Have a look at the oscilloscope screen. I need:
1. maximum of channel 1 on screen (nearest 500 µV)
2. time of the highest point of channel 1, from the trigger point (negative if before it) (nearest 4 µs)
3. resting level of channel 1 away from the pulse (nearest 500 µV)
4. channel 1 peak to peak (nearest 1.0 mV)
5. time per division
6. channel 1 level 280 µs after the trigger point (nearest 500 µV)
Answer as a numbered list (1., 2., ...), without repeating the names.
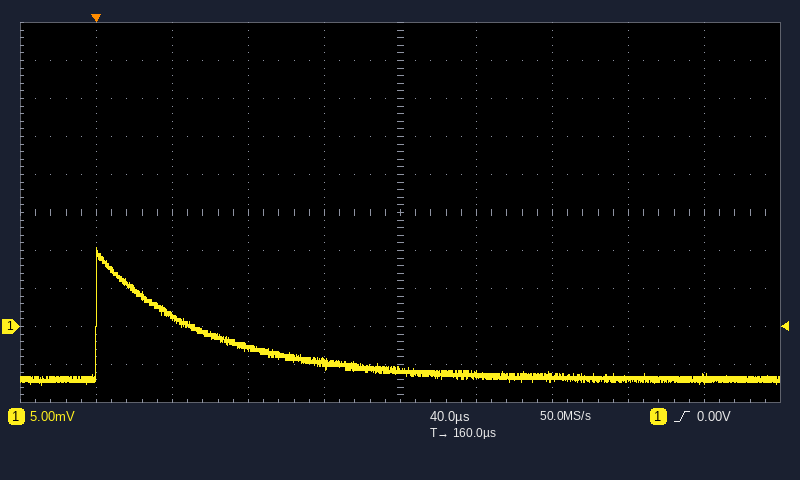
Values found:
1. 10.5 mV
2. 0 µs
3. -7.0 mV
4. 18.0 mV
5. 40 µs
6. -7.0 mV
